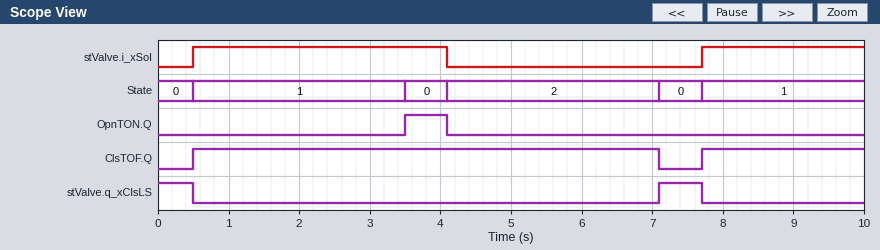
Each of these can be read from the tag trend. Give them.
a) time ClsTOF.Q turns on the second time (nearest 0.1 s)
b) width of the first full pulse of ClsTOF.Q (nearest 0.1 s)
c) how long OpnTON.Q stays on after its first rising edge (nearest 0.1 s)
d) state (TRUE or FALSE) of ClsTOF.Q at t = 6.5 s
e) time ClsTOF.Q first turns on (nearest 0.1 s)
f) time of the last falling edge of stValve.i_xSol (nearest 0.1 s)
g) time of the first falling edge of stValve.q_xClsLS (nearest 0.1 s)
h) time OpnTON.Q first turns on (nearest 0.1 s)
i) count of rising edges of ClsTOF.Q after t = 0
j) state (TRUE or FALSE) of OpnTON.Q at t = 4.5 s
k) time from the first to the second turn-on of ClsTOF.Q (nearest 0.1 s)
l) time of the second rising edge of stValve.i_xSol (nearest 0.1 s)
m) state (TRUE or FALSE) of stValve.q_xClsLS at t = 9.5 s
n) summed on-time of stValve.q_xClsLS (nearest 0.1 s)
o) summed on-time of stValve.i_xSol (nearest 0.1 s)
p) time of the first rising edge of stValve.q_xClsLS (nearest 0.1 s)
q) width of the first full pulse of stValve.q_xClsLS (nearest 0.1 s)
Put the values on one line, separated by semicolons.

7.7 s; 6.6 s; 0.6 s; TRUE; 0.5 s; 4.1 s; 0.5 s; 3.5 s; 2; FALSE; 7.2 s; 7.7 s; FALSE; 1.1 s; 5.9 s; 7.1 s; 0.6 s
